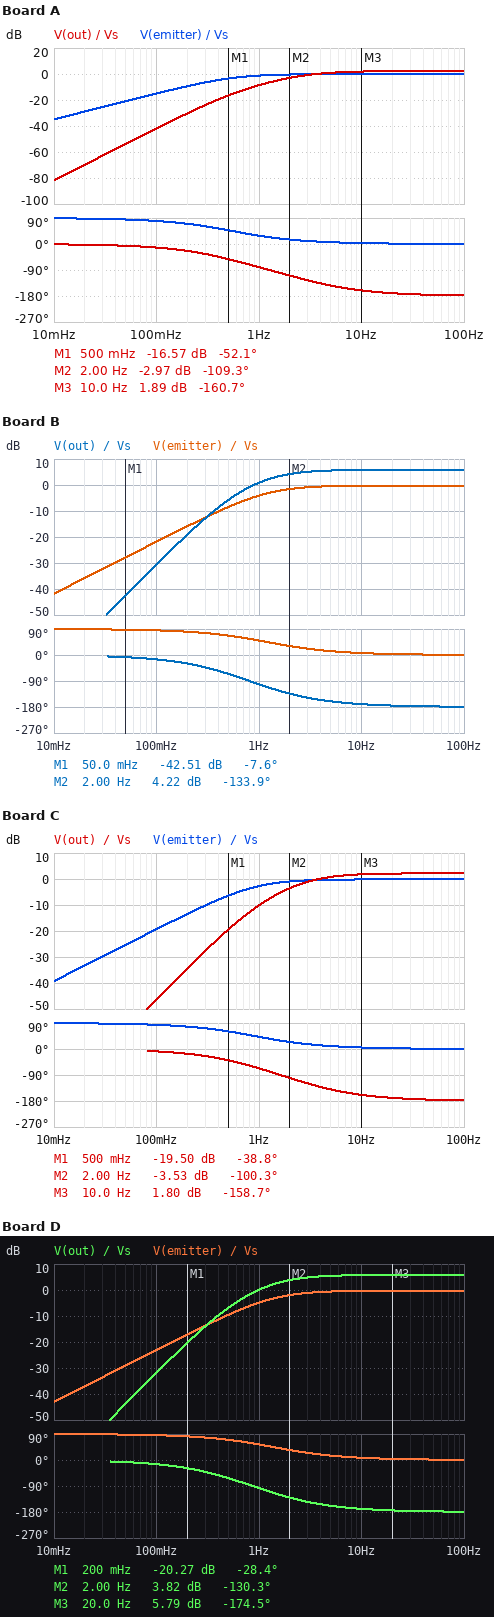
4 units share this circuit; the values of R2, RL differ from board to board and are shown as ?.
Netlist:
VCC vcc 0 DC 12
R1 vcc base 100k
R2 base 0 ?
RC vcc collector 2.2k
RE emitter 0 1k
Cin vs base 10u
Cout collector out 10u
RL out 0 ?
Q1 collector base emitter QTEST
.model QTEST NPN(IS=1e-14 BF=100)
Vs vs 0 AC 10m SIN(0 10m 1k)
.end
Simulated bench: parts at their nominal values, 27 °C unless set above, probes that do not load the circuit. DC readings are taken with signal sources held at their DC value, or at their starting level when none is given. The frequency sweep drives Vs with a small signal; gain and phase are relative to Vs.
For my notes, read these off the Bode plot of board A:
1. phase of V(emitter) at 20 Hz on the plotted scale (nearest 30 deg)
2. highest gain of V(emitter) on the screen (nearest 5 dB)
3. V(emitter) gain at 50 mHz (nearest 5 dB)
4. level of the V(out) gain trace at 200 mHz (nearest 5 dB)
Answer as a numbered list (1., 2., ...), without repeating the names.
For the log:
1. 0 deg
2. 0 dB
3. -20 dB
4. -30 dB
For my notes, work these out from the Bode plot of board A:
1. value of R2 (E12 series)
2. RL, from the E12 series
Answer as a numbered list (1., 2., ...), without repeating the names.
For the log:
1. 68 kΩ
2. 3.3 kΩ
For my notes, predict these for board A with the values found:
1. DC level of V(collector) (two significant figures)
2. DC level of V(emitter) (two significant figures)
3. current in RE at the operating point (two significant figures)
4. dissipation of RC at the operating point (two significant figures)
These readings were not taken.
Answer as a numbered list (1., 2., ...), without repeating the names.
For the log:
1. 5.5 V
2. 3.0 V
3. 3.0 mA
4. 19 mW
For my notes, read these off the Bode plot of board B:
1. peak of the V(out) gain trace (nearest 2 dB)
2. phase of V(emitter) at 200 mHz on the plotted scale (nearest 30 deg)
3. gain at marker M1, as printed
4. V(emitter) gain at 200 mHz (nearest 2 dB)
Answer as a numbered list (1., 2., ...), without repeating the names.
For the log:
1. 6 dB
2. 90 deg
3. -42.51 dB
4. -16 dB
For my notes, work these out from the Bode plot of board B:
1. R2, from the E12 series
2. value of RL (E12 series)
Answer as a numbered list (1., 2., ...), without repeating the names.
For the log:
1. 18 kΩ
2. 27 kΩ
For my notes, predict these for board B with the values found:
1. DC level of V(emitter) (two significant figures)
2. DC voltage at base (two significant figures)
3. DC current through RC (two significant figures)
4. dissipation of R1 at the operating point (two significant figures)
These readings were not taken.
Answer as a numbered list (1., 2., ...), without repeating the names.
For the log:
1. 1.0 V
2. 1.7 V
3. 1.0 mA
4. 1.1 mW
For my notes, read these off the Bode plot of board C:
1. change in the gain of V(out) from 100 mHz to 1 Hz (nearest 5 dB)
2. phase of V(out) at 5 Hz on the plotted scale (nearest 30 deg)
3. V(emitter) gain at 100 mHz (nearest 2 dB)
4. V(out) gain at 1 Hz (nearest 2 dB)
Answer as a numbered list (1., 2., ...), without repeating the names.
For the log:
1. 35 dB
2. -150 deg
3. -20 dB
4. -10 dB
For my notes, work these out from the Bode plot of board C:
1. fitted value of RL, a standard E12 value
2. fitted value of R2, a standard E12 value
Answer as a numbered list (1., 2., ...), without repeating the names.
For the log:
1. 3.3 kΩ
2. 27 kΩ
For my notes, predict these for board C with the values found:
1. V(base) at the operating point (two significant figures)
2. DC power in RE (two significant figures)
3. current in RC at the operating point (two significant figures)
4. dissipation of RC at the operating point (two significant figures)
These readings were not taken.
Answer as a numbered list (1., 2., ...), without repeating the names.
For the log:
1. 2.2 V
2. 2.4 mW
3. 1.5 mA
4. 5.2 mW
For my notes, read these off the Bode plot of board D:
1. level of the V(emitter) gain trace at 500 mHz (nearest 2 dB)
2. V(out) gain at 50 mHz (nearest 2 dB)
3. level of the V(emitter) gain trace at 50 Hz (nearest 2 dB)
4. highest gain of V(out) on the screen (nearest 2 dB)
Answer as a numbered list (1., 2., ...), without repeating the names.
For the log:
1. -10 dB
2. -44 dB
3. 0 dB
4. 6 dB
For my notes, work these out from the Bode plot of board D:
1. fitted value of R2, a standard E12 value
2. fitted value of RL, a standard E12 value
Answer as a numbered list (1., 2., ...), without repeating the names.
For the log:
1. 15 kΩ
2. 27 kΩ
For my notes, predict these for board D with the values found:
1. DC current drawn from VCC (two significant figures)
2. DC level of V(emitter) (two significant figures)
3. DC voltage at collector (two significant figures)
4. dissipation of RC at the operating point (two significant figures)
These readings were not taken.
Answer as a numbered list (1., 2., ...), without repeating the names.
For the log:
1. 910 µA
2. 810 mV
3. 10 V
4. 1.4 mW
